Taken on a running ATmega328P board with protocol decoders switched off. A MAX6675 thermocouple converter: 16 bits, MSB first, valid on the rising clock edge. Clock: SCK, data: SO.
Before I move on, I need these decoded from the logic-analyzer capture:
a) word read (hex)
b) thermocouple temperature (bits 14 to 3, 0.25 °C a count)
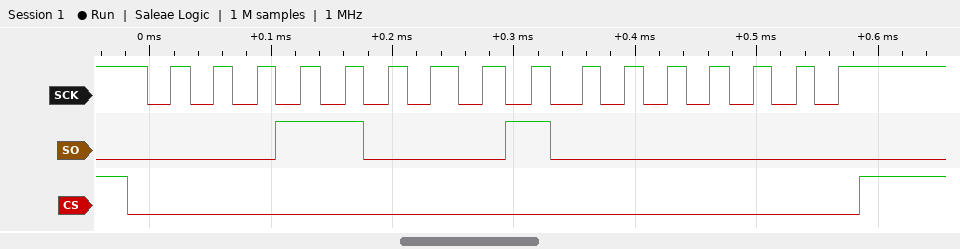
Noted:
0x1880
196.00 °C
